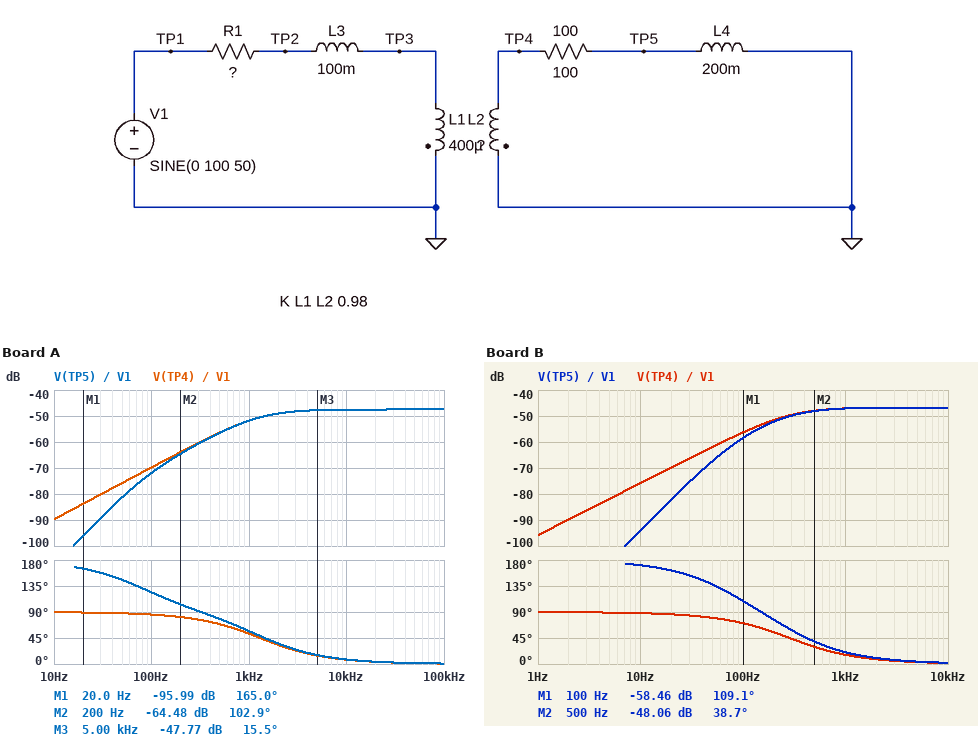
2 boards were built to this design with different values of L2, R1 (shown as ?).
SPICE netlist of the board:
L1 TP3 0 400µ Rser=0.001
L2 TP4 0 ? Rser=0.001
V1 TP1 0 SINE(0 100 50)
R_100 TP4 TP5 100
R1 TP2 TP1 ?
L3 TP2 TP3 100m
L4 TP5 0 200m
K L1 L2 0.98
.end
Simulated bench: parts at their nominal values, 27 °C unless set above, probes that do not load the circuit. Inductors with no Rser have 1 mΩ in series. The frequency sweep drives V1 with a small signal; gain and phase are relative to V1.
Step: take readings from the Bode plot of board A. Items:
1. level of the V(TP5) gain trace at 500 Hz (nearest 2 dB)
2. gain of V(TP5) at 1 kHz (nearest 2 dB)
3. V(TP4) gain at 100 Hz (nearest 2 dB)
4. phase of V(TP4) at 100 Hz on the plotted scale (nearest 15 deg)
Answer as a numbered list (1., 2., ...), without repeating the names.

1. -56 dB
2. -52 dB
3. -70 dB
4. 90 deg
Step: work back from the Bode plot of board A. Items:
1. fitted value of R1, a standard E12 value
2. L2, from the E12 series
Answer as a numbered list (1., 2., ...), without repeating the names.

1. 820 Ω
2. 470 µH
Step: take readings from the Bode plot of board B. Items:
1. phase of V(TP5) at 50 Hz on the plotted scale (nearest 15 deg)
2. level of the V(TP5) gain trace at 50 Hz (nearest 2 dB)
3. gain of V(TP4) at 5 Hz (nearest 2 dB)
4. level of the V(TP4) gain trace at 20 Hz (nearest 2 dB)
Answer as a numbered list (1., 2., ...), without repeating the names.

1. 135 deg
2. -68 dB
3. -82 dB
4. -70 dB
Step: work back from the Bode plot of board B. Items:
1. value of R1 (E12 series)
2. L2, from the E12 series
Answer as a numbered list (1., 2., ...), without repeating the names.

1. 180 Ω
2. 560 µH
